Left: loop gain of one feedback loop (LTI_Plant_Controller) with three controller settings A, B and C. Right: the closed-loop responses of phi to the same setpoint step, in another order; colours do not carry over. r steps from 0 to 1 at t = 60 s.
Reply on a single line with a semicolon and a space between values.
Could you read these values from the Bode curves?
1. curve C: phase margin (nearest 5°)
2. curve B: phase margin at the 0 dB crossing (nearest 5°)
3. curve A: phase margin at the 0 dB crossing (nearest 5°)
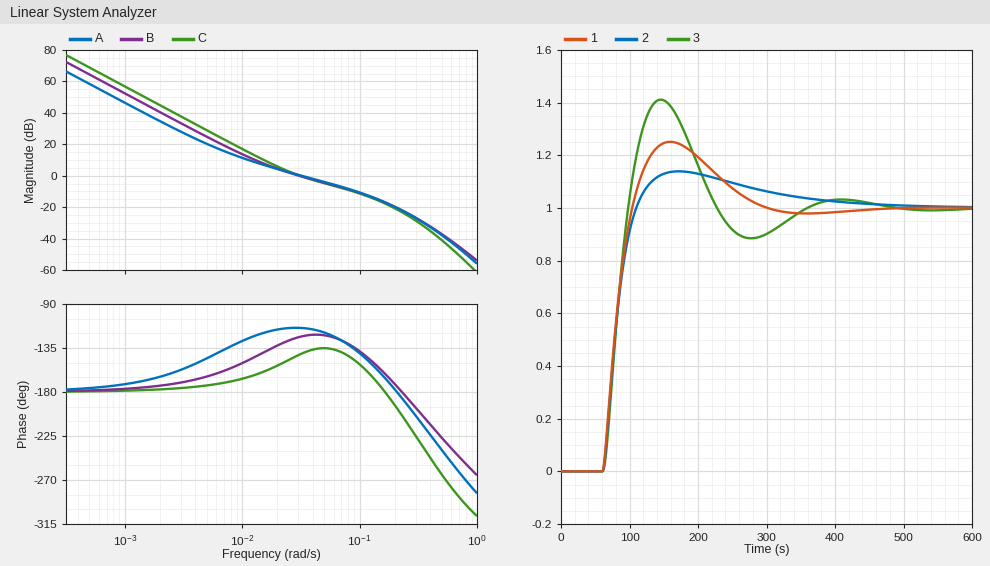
40°; 55°; 65°
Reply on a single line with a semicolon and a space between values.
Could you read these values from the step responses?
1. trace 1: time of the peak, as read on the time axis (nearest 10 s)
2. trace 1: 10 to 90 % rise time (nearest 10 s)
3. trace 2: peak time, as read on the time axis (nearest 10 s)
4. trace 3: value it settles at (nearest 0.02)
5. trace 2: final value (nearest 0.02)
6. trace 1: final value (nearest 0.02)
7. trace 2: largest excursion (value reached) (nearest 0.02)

160 s; 30 s; 170 s; 1.00; 1.00; 1.00; 1.14
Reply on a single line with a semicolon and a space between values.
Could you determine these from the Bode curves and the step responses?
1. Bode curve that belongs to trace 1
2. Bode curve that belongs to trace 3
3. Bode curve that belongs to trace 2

B; C; A
